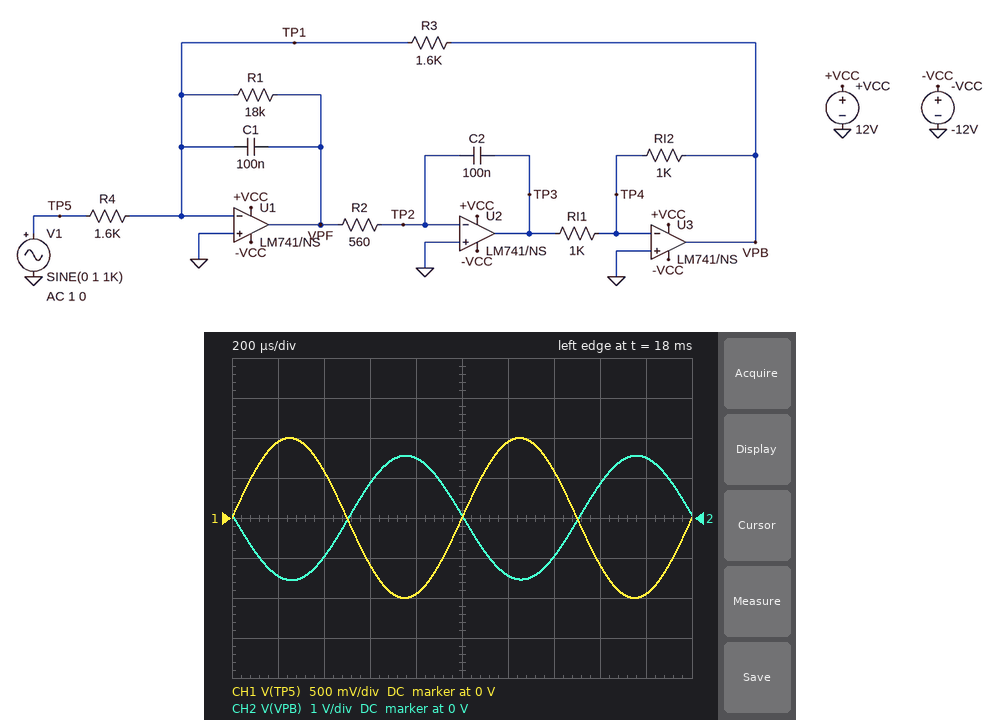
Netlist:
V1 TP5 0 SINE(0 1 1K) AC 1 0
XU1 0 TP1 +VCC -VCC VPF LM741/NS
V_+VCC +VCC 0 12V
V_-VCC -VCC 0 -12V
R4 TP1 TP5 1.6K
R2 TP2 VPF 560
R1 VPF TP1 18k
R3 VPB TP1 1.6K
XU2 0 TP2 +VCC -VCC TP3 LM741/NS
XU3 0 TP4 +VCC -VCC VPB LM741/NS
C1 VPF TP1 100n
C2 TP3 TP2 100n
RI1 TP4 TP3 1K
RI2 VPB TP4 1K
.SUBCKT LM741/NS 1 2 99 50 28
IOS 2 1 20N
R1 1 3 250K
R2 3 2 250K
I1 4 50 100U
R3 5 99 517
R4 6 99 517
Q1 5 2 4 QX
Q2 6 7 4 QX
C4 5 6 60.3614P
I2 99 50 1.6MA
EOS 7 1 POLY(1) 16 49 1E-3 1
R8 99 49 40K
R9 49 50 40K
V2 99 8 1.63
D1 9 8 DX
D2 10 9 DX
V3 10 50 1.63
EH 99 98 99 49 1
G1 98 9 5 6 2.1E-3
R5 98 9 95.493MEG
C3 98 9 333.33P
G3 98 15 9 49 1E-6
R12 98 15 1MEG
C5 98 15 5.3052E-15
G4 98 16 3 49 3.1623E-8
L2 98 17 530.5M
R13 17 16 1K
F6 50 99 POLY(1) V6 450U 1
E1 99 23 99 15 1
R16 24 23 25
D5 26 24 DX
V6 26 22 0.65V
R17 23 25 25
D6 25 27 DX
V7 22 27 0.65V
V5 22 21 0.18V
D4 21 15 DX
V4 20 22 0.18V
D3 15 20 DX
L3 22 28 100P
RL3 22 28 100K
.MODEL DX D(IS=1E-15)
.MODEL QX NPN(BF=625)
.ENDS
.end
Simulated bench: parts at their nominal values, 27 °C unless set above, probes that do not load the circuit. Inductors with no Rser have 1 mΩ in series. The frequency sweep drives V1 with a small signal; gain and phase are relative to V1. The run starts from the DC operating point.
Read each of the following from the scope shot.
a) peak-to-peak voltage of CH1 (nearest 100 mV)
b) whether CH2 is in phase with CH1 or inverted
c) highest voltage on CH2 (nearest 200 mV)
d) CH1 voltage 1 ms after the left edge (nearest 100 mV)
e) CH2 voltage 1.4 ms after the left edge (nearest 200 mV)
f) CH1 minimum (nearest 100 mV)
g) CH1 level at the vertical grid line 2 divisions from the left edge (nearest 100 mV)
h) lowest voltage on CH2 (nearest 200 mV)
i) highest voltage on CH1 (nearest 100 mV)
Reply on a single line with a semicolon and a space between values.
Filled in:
2.0 V; inverted; 1.6 V; 0 V; -1.0 V; -1.0 V; 600 mV; -1.6 V; 1.0 V
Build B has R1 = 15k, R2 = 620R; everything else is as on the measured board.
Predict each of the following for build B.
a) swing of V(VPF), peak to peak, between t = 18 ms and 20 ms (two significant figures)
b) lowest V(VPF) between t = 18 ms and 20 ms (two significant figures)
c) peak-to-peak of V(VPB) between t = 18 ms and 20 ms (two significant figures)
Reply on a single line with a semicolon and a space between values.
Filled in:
1.3 V; -640 mV; 3.3 V
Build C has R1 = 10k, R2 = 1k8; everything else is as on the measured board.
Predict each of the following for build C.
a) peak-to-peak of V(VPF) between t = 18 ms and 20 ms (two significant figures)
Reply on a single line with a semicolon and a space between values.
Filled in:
10 V
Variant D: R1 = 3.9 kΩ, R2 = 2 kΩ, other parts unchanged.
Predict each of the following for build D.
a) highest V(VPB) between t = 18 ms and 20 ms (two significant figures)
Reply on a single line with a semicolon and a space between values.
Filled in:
1.7 V
